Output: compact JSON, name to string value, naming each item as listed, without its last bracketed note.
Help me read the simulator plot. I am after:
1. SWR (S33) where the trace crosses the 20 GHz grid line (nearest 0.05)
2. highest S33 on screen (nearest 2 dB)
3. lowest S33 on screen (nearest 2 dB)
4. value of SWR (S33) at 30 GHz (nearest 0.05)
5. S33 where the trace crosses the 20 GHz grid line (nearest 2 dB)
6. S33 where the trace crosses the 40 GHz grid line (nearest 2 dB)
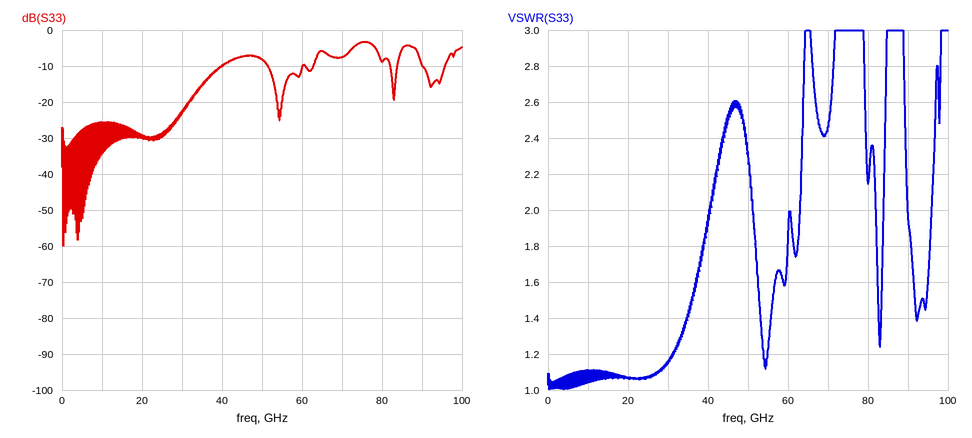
{"SWR (S33) where the trace crosses the 20 GHz grid line": "1.05", "highest S33 on screen": "-4 dB", "lowest S33 on screen": "-60 dB", "value of SWR (S33) at 30 GHz": "1.15", "S33 where the trace crosses the 20 GHz grid line": "-30 dB", "S33 where the trace crosses the 40 GHz grid line": "-10 dB"}
